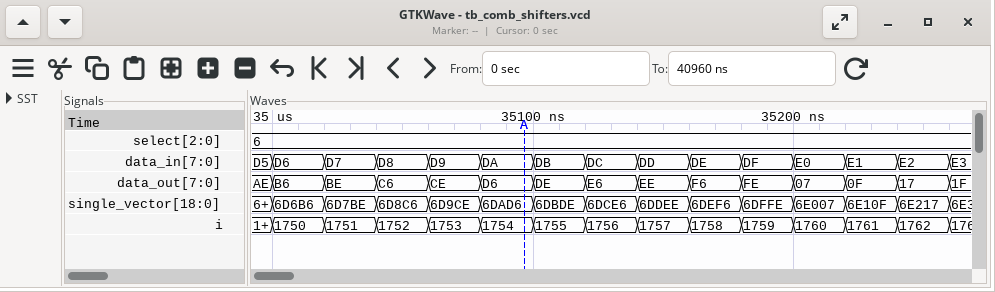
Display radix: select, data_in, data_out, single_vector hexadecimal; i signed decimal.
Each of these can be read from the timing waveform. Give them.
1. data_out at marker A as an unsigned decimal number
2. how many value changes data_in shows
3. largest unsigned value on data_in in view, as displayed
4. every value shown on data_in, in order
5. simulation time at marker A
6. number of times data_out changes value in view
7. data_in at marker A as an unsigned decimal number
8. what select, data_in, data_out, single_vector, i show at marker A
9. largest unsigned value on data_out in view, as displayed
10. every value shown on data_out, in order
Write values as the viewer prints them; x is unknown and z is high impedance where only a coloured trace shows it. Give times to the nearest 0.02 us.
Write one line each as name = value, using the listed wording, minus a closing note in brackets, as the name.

data_out at marker A as an unsigned decimal number = 214
how many value changes data_in shows = 14
largest unsigned value on data_in in view, as displayed = E3
every value shown on data_in, in order = D5, D6, D7, D8, D9, DA, DB, DC, DD, DE, DF, E0, E1, E2, E3
simulation time at marker A = 35.1 us
number of times data_out changes value in view = 14
data_in at marker A as an unsigned decimal number = 218
what select, data_in, data_out, single_vector, i show at marker A = select=6, data_in=DA, data_out=D6, single_vector=6DAD6, i=1754
largest unsigned value on data_out in view, as displayed = FE
every value shown on data_out, in order = AE, B6, BE, C6, CE, D6, DE, E6, EE, F6, FE, 07, 0F, 17, 1F
